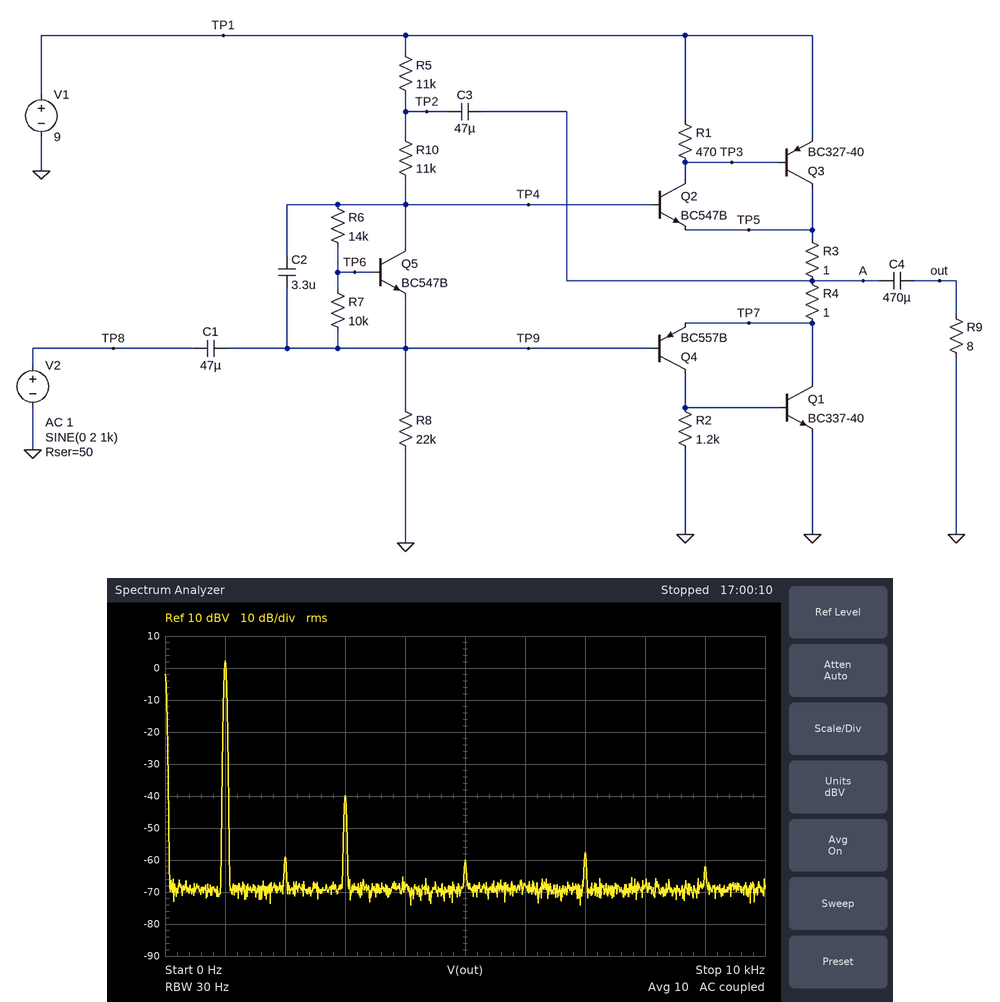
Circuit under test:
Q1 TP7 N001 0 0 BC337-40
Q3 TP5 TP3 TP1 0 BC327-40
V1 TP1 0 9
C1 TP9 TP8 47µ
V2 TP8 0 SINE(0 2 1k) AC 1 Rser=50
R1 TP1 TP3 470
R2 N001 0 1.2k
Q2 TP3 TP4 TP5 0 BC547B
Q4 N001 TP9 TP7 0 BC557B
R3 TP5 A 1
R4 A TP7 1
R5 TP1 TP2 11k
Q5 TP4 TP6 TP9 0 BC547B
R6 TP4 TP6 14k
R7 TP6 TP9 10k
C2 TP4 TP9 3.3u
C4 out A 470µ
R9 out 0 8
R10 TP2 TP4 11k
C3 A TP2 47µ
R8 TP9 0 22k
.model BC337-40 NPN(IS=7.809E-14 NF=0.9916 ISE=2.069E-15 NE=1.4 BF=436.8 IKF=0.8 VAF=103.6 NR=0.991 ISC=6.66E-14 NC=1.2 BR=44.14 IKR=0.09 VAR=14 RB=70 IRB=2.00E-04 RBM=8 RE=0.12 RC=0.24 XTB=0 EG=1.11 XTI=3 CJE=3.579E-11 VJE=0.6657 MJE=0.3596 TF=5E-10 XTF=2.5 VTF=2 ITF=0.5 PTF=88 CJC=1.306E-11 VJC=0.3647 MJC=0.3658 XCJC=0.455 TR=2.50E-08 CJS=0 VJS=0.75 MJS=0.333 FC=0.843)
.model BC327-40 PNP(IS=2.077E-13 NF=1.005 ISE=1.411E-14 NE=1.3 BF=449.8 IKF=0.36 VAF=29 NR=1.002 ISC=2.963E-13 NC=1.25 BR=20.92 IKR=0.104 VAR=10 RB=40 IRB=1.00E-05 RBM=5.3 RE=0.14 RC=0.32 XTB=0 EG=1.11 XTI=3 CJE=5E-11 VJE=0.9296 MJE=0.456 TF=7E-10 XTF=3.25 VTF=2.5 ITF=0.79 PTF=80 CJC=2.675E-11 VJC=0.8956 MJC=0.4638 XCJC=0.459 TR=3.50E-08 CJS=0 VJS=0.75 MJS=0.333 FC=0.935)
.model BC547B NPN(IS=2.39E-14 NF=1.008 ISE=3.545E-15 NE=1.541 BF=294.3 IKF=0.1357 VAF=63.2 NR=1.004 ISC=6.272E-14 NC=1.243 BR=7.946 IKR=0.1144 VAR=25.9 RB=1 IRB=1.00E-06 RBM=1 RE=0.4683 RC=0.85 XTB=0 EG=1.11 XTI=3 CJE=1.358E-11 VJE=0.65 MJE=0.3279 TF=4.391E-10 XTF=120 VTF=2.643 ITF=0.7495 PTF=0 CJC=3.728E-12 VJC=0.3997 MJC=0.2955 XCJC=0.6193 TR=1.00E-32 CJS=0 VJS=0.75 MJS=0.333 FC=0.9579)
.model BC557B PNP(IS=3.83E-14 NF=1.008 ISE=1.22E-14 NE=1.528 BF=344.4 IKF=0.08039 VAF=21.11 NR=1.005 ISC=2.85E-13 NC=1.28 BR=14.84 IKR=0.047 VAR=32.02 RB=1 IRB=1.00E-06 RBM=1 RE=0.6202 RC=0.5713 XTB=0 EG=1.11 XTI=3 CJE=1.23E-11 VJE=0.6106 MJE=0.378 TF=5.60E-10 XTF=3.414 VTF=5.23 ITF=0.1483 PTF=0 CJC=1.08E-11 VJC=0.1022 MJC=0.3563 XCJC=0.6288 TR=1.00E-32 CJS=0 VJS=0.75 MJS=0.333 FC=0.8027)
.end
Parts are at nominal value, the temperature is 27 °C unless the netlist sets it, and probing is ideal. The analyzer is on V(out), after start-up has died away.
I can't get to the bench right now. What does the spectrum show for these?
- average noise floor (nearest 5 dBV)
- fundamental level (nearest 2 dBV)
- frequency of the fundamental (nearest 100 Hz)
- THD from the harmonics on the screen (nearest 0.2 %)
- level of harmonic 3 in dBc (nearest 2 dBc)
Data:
-70 dBV
2 dBV
1.0 kHz
0.8 %
-42 dBc
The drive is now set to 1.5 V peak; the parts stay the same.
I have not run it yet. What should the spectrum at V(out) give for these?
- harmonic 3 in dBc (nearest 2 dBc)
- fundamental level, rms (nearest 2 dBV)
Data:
-46 dBc
0 dBV
